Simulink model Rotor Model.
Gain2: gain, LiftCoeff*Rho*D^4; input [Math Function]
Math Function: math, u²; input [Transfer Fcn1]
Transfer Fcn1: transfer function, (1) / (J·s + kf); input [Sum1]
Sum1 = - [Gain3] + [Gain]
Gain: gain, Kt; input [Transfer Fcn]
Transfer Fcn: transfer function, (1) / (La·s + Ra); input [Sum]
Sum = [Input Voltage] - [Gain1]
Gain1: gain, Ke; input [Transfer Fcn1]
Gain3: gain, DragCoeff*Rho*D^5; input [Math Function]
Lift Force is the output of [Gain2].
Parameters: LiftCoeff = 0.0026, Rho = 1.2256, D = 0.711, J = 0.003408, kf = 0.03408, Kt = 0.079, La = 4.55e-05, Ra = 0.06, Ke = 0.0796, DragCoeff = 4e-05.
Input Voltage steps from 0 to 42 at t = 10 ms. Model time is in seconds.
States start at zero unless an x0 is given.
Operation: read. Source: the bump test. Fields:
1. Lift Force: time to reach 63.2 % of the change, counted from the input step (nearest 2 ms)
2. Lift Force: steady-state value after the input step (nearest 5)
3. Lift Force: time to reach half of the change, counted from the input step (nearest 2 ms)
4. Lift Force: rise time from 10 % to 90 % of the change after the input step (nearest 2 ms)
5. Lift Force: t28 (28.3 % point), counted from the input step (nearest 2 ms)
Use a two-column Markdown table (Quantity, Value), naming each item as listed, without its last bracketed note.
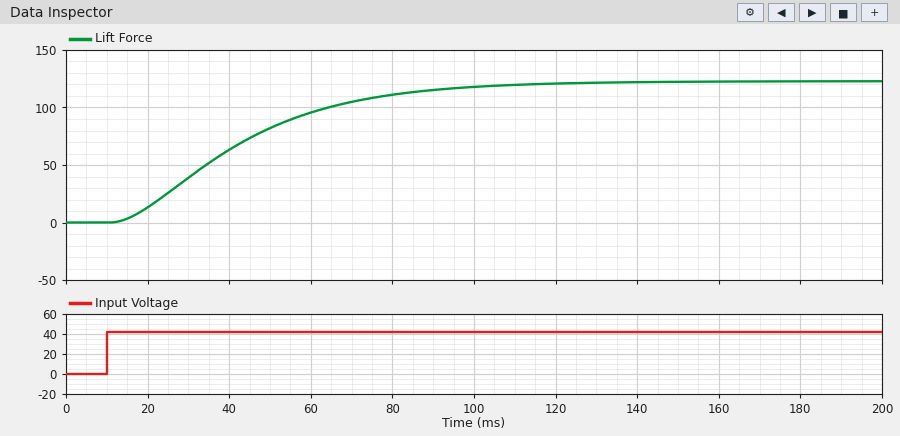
| Quantity | Value |
|---|---|
| Lift Force: time to reach 63.2 % of the change, counted from the input step | 38 ms |
| Lift Force: steady-state value after the input step | 125 |
| Lift Force: time to reach half of the change, counted from the input step | 30 ms |
| Lift Force: rise time from 10 % to 90 % of the change after the input step | 60 ms |
| Lift Force: t28 (28.3 % point), counted from the input step | 18 ms |
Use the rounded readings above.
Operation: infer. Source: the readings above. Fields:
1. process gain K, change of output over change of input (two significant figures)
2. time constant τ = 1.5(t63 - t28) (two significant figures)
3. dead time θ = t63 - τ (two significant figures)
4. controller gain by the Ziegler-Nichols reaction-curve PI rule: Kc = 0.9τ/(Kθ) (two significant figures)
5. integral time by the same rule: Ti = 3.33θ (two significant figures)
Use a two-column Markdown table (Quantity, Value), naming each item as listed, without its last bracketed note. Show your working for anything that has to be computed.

| Quantity | Value |
|---|---|
| process gain K, change of output over change of input | (125 - 0) / 42 = 3.0 |
| time constant τ = 1.5(t63 - t28) | 1.5 × (38 - 18) = 30 ms |
| dead time θ = t63 - τ | 38 - 30 = 8.0 ms |
| controller gain by the Ziegler-Nichols reaction-curve PI rule: Kc = 0.9τ/(Kθ) | 0.9 × 30 / (3 × 8) = 1.1 |
| integral time by the same rule: Ti = 3.33θ | 3.33 × 8 = 27 ms |
